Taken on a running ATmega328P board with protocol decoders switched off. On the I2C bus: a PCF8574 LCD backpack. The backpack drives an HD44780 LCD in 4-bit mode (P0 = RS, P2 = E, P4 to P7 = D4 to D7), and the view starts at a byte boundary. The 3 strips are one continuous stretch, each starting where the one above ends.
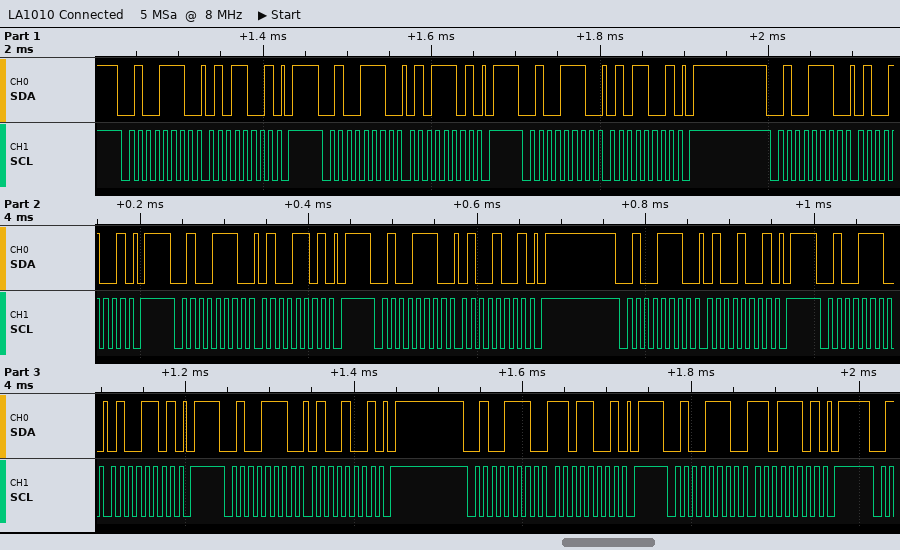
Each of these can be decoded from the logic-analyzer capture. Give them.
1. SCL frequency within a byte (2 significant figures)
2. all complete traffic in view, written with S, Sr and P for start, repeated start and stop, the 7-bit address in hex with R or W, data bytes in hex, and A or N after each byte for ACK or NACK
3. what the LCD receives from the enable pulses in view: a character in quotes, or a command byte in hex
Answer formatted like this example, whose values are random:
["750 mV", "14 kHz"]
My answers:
["100 kHz", "S 27W A 59 A P S 27W A 5D A P S 27W A 59 A P S 27W A 49 A P S 27W A 4D A P S 27W A 49 A P S 27W A 49 A P S 27W A 4D A P S 27W A 49 A P S 27W A D9 A P S 27W A DD A P", "'T'"]
